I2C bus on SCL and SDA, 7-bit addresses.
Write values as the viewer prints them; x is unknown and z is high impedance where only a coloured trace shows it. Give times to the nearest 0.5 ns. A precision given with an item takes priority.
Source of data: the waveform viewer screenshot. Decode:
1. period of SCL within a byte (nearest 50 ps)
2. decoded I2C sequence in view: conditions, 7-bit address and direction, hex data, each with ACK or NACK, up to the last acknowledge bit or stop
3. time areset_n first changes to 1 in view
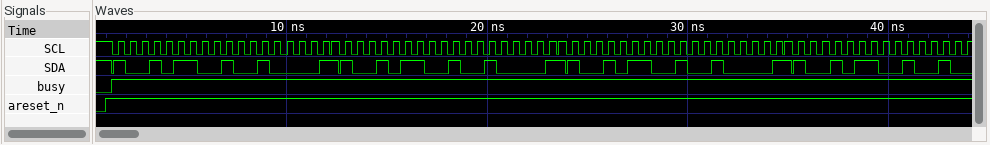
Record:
600 ps
start, address 4B write ACK, 90 NACK, repeated start, address 4B write ACK, 90 NACK, repeated start, address 4B write ACK, 90 NACK, repeated start, address 4B write ACK
1 ns
